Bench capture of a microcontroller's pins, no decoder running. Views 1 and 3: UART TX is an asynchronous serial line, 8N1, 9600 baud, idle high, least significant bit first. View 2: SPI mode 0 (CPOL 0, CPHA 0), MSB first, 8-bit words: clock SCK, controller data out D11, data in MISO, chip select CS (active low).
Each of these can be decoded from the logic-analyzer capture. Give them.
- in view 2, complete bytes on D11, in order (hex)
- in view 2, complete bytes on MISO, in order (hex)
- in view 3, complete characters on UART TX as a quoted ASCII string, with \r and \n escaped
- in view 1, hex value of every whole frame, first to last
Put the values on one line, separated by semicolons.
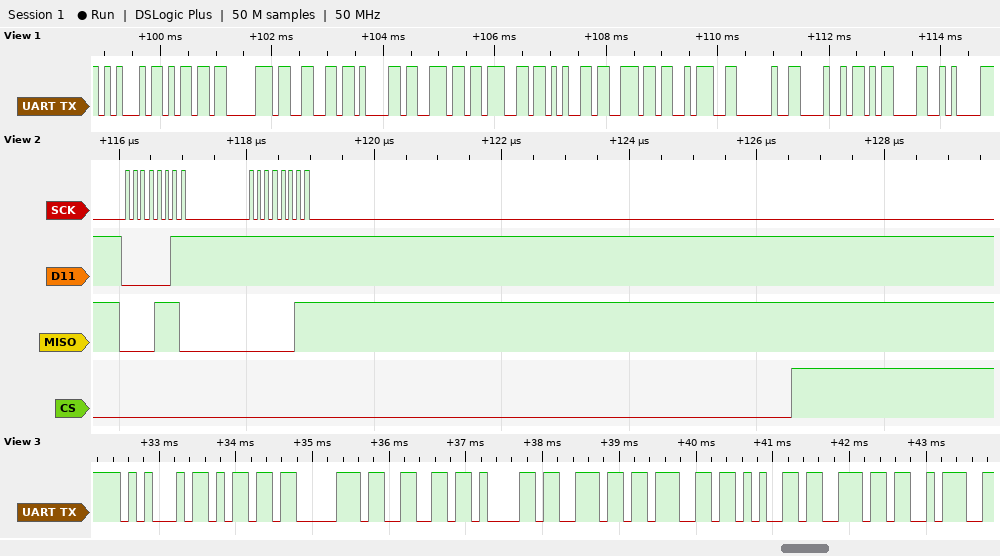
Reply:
03 FF; 0E 03; "Empfangen:"; 0x45 0x6D 0x70 0x66 0x61 0x6E 0x67 0x65 0x6E 0x3A 0x20 0x48 0x0D 0x0A
